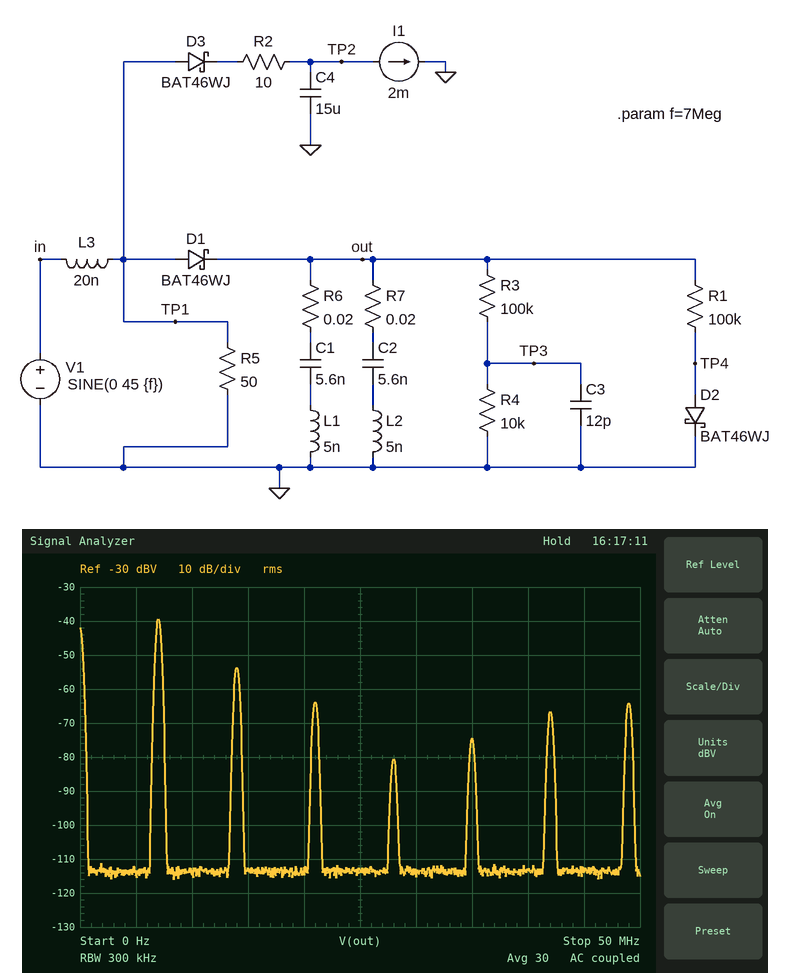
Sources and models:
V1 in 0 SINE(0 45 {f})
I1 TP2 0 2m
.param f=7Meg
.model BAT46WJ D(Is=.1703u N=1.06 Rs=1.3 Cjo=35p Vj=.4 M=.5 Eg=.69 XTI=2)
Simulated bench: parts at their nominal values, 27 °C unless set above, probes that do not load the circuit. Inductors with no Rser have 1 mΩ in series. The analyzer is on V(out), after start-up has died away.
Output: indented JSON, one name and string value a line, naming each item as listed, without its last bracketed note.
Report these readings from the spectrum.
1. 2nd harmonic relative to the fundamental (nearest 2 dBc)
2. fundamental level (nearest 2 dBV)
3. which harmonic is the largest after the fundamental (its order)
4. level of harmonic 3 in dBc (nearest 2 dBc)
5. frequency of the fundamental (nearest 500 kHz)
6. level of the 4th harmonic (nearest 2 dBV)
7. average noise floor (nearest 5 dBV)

{
  "2nd harmonic relative to the fundamental": "-14 dBc",
  "fundamental level": "-40 dBV",
  "which harmonic is the largest after the fundamental": "2",
  "level of harmonic 3 in dBc": "-24 dBc",
  "frequency of the fundamental": "7.0 MHz",
  "level of the 4th harmonic": "-80 dBV",
  "average noise floor": "-115 dBV"
}
